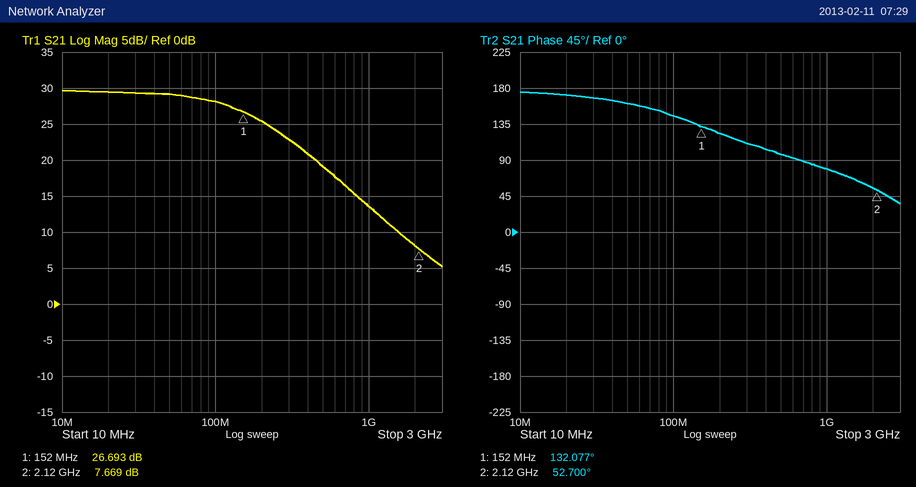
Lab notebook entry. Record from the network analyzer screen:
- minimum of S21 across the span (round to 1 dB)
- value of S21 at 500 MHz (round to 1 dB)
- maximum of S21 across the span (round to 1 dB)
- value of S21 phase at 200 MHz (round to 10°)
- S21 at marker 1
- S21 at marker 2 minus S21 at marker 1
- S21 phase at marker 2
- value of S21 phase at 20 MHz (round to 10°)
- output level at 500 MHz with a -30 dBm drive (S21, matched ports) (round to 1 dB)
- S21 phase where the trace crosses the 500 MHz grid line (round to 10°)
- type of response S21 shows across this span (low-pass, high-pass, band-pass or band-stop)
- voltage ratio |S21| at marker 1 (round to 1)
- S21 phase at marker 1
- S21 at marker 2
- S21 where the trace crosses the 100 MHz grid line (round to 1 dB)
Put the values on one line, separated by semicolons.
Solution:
5 dB; 19 dB; 30 dB; 120°; 26.693 dB; -19.024 dB; 52.700°; 170°; -11 dBm; 100°; low-pass; 22; 132.077°; 7.669 dB; 28 dB
